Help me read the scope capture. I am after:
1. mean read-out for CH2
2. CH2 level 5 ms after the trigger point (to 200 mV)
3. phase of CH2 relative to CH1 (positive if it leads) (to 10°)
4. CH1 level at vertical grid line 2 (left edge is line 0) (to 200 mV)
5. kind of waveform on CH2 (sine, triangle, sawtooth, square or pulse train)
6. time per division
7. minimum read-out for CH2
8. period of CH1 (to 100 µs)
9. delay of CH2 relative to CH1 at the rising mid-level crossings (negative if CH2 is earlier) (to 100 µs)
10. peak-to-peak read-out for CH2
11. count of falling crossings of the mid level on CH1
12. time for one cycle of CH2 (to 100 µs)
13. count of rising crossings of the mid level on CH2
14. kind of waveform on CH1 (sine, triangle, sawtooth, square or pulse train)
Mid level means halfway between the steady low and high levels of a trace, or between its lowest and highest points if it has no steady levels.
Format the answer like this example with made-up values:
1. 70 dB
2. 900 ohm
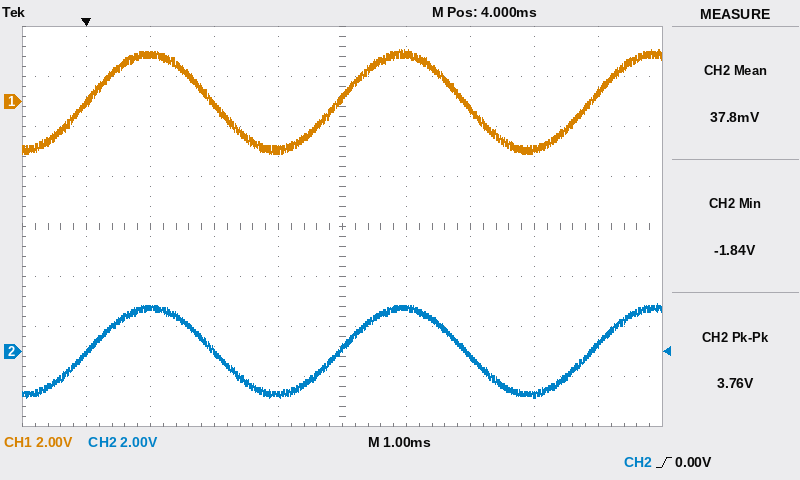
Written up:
1. 37.8 mV
2. 1.8 V
3. 0°
4. 1.8 V
5. sine
6. 1 ms
7. -1.84 V
8. 3.9 ms
9. 0.0 ms
10. 3.76 V
11. 2
12. 3.9 ms
13. 3
14. sine
